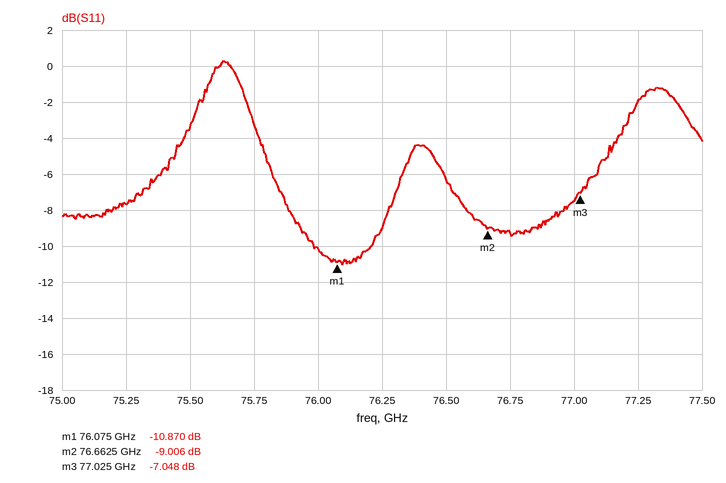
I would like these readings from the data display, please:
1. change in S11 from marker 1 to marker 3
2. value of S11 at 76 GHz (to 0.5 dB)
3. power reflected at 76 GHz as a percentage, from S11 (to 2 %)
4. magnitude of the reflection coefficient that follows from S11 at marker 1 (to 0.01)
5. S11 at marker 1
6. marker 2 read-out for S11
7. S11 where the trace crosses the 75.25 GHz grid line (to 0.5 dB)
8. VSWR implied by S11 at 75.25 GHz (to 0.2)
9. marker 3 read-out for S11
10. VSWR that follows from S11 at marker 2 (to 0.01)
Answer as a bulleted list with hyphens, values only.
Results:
- 3.822 dB
- -10.0 dB
- 10 %
- 0.29
- -10.870 dB
- -9.006 dB
- -7.5 dB
- 2.4
- -7.048 dB
- 2.10
